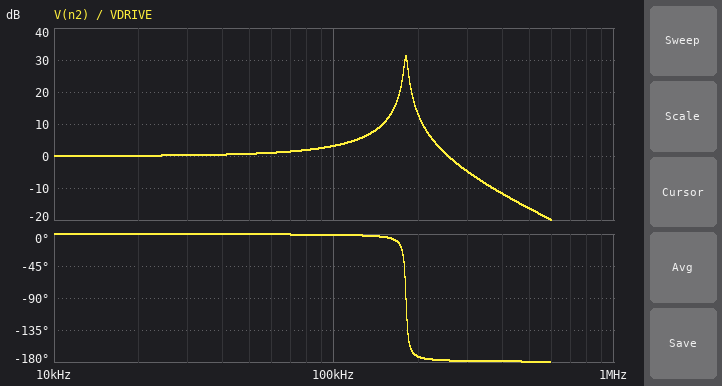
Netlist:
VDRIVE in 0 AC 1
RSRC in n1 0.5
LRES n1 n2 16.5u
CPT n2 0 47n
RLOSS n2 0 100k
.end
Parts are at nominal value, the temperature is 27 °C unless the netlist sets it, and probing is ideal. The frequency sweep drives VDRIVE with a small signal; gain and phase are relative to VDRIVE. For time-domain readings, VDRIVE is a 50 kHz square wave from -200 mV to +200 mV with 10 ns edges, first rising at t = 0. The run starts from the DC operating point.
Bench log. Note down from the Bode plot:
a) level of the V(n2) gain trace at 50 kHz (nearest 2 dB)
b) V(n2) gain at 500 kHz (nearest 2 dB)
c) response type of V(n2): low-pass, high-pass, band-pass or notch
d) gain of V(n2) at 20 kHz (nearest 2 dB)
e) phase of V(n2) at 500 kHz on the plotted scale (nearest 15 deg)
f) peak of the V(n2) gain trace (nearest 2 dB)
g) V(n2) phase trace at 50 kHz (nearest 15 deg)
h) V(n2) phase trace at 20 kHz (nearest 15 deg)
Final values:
0 dB
-16 dB
low-pass
0 dB
-180 deg
32 dB
0 deg
0 deg
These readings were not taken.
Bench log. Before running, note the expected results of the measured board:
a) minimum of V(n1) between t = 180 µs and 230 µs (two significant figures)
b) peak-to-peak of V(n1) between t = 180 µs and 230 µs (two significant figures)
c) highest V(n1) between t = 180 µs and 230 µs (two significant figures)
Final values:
-210 mV
410 mV
210 mV
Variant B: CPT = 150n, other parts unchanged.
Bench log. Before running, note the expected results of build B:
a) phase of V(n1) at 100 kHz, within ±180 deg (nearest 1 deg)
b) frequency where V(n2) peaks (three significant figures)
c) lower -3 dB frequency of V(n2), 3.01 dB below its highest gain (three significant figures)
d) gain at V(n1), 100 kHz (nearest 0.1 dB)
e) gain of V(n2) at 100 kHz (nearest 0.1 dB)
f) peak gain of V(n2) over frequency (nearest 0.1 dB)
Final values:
-64 deg
101 kHz
98.7 kHz
-7.2 dB
25.6 dB
26.4 dB
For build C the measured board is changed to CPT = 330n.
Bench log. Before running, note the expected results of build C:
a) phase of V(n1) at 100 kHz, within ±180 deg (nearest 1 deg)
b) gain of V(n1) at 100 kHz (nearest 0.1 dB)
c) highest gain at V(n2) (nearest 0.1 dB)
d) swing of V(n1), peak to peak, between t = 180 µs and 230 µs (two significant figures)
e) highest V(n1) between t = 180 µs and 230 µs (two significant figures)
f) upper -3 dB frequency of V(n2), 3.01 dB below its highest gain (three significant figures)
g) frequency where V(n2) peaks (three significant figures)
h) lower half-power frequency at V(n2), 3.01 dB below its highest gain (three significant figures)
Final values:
5 deg
0 dB
23.0 dB
450 mV
230 mV
70.5 kHz
68.1 kHz
65.7 kHz
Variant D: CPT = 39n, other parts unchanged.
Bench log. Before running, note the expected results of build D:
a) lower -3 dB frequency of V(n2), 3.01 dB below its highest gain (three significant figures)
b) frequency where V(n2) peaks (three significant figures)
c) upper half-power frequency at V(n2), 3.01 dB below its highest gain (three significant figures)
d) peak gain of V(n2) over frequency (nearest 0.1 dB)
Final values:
196 kHz
198 kHz
201 kHz
32.2 dB
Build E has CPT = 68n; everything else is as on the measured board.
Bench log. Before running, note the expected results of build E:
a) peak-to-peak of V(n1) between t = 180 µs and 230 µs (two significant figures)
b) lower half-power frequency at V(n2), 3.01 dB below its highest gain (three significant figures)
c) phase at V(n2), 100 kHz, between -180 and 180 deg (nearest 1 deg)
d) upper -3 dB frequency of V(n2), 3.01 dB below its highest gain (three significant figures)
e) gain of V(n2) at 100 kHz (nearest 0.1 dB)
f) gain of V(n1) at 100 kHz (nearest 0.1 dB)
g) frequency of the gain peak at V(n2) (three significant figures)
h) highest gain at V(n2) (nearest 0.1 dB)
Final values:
560 mV
148 kHz
-2 deg
153 kHz
5.1 dB
0 dB
150 kHz
29.8 dB
